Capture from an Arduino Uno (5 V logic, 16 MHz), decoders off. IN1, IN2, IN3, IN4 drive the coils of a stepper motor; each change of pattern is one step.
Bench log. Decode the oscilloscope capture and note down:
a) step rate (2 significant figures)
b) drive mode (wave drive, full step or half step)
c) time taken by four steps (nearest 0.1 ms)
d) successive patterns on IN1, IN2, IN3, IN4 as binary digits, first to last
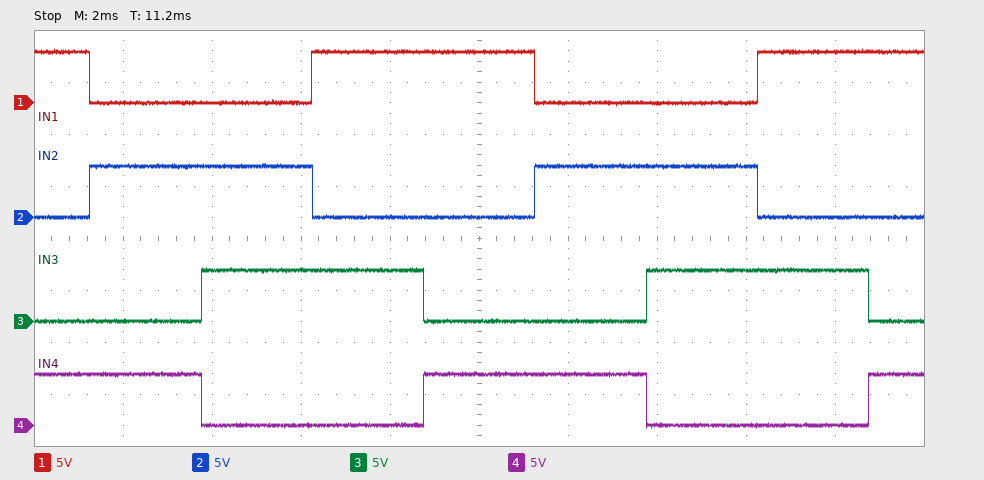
400 steps/s
full step
10.0 ms
1001 0101 0110 1010 1001 0101 0110 1010 1001
